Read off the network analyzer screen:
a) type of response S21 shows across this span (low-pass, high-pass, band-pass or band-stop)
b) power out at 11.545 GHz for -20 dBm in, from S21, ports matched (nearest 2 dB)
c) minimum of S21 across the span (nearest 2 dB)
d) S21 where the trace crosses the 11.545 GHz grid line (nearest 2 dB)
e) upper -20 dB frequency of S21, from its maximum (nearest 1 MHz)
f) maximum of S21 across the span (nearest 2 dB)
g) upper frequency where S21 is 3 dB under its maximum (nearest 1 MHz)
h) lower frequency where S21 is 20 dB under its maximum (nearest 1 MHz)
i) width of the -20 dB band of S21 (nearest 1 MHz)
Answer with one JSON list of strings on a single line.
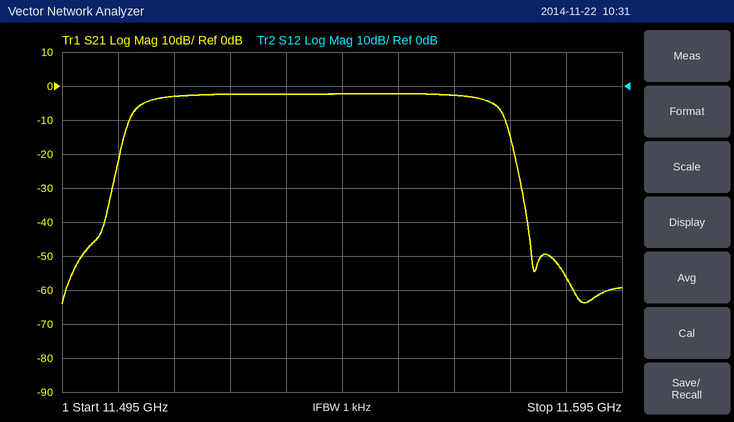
["band-pass", "-22 dBm", "-64 dB", "-2 dB", "11.576 GHz", "-2 dB", "11.572 GHz", "11.505 GHz", "71 MHz"]
